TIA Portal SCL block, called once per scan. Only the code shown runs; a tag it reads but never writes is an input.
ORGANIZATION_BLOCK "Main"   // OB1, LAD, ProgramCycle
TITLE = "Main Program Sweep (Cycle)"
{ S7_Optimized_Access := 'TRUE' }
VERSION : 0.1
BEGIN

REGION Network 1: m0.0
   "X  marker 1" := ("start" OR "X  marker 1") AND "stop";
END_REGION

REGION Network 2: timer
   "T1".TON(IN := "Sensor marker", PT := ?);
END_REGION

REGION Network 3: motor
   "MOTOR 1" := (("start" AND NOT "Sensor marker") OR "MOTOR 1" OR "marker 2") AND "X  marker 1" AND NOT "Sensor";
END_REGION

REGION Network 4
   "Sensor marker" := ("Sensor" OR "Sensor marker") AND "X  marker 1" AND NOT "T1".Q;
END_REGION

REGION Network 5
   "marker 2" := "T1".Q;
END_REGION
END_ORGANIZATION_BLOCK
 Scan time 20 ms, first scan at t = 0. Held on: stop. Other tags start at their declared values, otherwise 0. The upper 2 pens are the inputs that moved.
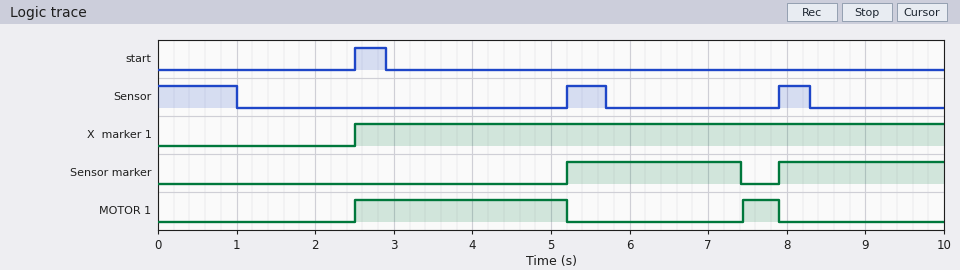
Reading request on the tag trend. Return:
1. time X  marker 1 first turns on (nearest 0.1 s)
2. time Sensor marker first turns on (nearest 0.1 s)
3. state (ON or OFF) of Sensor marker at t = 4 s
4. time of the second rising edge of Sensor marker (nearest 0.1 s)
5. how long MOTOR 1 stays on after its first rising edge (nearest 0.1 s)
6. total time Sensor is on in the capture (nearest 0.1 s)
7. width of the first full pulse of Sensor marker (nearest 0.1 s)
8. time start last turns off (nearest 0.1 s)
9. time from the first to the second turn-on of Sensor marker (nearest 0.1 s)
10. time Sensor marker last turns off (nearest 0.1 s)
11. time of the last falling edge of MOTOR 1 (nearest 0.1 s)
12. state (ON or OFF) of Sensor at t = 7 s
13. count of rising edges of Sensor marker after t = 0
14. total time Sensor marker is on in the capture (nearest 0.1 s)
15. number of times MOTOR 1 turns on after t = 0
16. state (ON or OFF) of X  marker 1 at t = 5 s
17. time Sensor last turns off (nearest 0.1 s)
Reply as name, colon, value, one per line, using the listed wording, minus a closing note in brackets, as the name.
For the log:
time X  marker 1 first turns on: 2.5 s
time Sensor marker first turns on: 5.2 s
state (ON or OFF) of Sensor marker at t = 4 s: OFF
time of the second rising edge of Sensor marker: 7.9 s
how long MOTOR 1 stays on after its first rising edge: 2.7 s
total time Sensor is on in the capture: 1.9 s
width of the first full pulse of Sensor marker: 2.2 s
time start last turns off: 2.9 s
time from the first to the second turn-on of Sensor marker: 2.7 s
time Sensor marker last turns off: 7.4 s
time of the last falling edge of MOTOR 1: 7.9 s
state (ON or OFF) of Sensor at t = 7 s: OFF
count of rising edges of Sensor marker after t = 0: 2
total time Sensor marker is on in the capture: 4.3 s
number of times MOTOR 1 turns on after t = 0: 2
state (ON or OFF) of X  marker 1 at t = 5 s: ON
time Sensor last turns off: 8.3 s
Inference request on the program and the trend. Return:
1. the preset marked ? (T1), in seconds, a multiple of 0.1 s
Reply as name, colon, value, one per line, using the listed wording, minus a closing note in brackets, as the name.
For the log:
the preset marked ? (T1), in seconds, a multiple of 0.1 s: 2.2 s
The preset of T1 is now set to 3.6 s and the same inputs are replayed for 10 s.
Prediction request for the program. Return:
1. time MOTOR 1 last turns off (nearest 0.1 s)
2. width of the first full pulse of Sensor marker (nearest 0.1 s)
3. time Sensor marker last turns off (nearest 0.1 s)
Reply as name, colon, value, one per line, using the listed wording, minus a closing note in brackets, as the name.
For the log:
time MOTOR 1 last turns off: 5.2 s
width of the first full pulse of Sensor marker: 3.6 s
time Sensor marker last turns off: 8.8 s
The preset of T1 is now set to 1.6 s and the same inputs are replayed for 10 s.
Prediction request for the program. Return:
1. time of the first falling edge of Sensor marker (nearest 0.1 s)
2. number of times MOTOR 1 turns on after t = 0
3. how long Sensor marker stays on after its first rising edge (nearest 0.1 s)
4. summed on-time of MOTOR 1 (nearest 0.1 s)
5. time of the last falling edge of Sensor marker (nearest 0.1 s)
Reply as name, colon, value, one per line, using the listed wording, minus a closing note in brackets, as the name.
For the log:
time of the first falling edge of Sensor marker: 6.8 s
number of times MOTOR 1 turns on after t = 0: 3
how long Sensor marker stays on after its first rising edge: 1.6 s
summed on-time of MOTOR 1: 4.2 s
time of the last falling edge of Sensor marker: 9.5 s
